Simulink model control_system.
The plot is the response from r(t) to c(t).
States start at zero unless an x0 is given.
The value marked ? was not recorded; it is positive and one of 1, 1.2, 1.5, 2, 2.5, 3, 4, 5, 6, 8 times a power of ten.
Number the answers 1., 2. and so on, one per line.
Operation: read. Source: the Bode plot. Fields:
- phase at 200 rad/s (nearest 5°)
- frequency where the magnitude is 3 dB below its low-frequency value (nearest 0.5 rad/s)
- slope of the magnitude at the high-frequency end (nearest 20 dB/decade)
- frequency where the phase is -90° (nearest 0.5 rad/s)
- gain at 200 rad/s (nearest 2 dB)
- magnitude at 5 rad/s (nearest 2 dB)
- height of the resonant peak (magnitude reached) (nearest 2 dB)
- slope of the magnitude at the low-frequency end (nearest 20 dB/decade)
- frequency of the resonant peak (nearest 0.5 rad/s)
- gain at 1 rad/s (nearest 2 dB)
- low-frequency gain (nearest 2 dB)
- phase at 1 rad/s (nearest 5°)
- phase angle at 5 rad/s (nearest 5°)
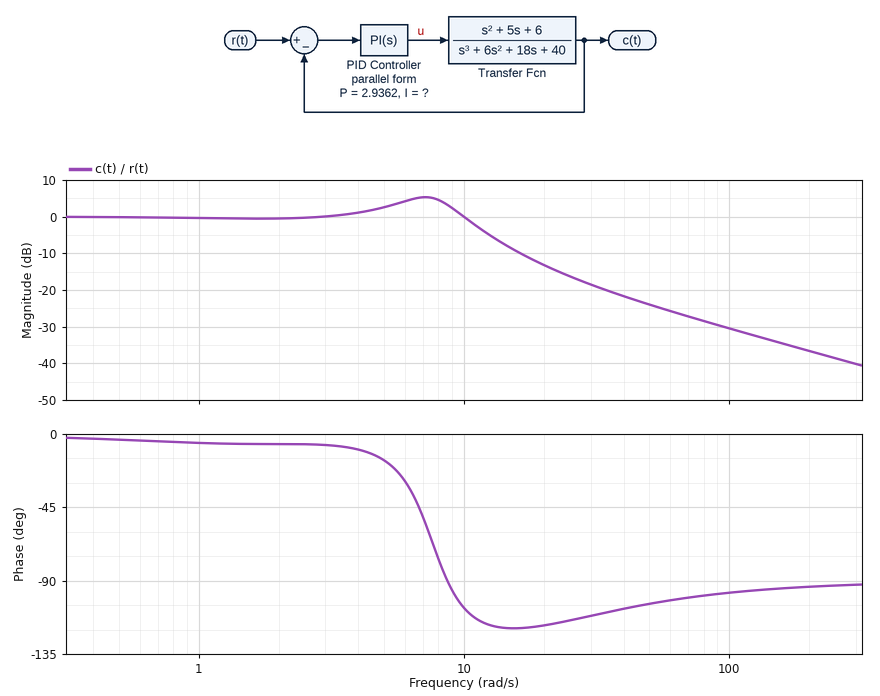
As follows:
1. -95°
2. 11.5 rad/s
3. -20 dB/decade
4. 8.5 rad/s
5. -36 dB
6. 2 dB
7. 6 dB
8. 0 dB/decade
9. 7.0 rad/s
10. 0 dB
11. 0 dB
12. -5°
13. -15°
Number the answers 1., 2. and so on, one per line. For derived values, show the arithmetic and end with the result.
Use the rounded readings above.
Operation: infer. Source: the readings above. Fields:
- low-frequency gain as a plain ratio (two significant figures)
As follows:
1. 10^(0 / 20) = 1.0
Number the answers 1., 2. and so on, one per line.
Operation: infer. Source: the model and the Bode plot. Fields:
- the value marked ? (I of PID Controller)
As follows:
1. 50
